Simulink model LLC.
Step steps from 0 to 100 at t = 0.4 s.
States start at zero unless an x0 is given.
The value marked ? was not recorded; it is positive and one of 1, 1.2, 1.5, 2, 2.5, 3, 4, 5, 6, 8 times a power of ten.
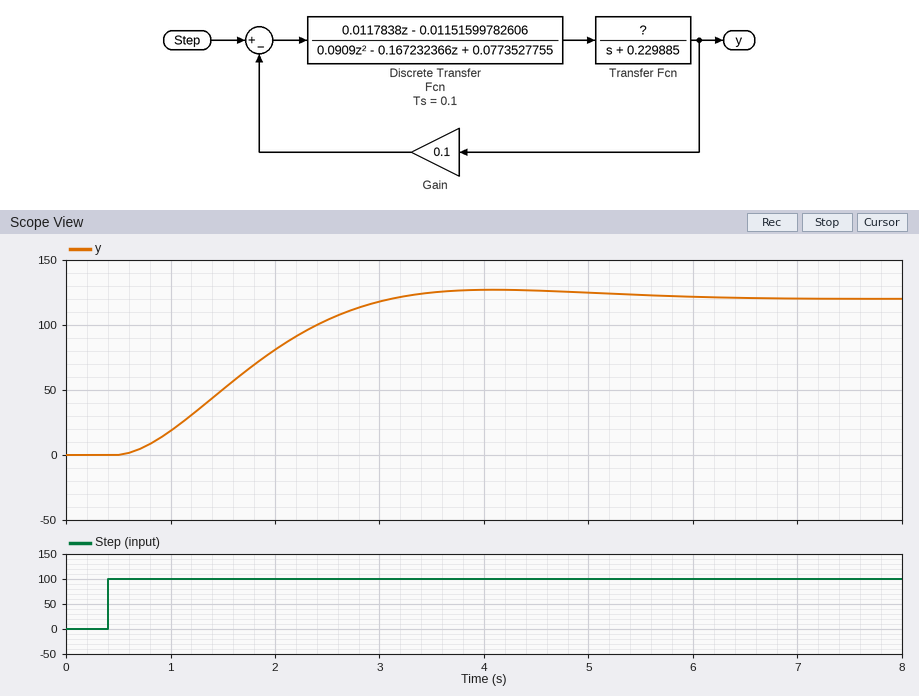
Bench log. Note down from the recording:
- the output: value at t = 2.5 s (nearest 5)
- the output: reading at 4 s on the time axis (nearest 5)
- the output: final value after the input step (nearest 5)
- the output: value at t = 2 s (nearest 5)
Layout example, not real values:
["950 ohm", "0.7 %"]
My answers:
["105", "125", "120", "80"]
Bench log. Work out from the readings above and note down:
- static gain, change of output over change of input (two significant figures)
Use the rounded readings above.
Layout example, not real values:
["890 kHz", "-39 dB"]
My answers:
["1.2"]
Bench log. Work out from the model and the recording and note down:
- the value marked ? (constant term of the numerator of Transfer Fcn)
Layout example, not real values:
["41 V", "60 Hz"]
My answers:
["1.2"]
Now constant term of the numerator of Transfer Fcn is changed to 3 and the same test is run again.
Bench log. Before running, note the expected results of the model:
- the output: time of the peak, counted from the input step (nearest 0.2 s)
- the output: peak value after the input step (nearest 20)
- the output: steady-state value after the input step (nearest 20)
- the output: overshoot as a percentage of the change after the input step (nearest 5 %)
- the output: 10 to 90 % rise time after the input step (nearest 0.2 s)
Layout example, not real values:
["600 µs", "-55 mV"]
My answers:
["3.2 s", "280", "260", "10 %", "1.4 s"]
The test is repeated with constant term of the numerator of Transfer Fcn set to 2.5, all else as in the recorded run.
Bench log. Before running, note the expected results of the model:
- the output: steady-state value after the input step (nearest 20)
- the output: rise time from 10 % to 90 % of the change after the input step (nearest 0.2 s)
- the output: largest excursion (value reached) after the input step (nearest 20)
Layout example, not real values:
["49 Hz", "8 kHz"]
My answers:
["220", "1.6 s", "240"]
